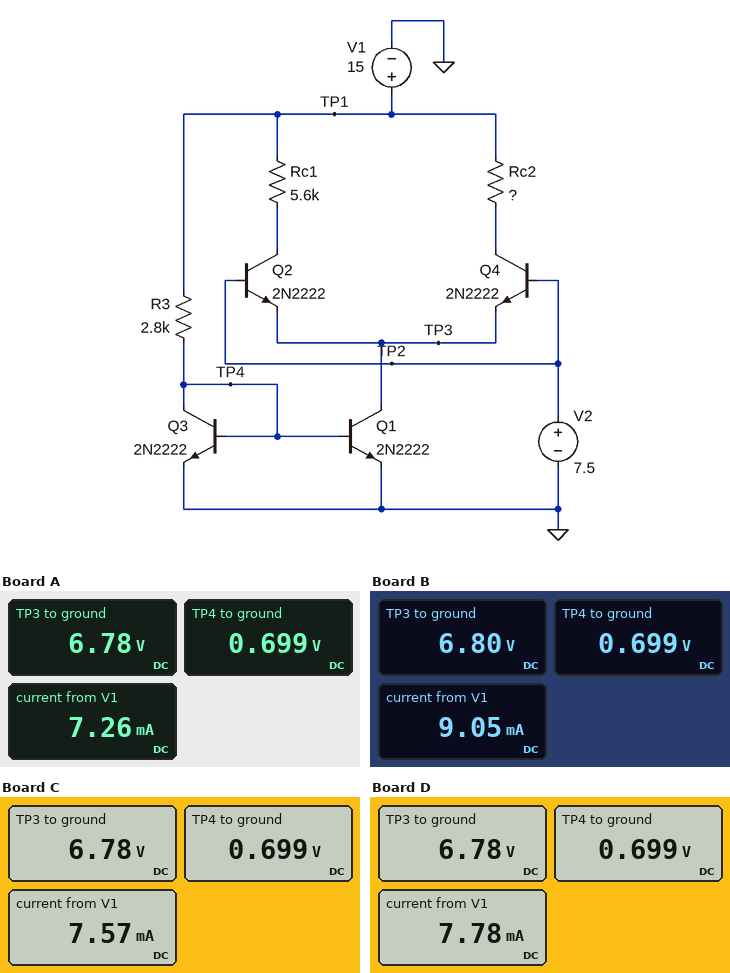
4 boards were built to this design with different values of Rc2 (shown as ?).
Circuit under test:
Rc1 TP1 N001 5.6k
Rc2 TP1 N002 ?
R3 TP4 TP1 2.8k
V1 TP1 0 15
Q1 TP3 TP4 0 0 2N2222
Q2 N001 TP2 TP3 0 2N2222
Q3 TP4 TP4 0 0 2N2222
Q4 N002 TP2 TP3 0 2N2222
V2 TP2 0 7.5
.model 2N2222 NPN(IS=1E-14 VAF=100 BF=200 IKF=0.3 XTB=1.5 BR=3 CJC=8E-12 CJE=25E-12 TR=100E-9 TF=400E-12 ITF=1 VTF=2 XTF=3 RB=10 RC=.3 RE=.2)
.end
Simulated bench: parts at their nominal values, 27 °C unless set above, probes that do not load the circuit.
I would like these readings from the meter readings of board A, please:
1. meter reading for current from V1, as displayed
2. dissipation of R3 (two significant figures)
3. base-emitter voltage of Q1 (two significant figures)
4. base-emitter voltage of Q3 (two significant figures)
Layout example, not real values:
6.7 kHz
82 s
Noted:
7.26 mA
73 mW
700 mV
700 mV
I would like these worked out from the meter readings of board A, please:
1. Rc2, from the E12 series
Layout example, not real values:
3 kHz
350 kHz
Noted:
12 kΩ
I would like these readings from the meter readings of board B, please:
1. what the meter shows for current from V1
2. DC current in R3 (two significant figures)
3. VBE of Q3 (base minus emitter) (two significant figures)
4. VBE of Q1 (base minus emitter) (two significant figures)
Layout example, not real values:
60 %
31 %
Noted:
9.05 mA
5.1 mA
700 mV
700 mV
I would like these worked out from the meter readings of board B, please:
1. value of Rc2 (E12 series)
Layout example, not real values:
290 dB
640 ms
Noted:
3.3 kΩ
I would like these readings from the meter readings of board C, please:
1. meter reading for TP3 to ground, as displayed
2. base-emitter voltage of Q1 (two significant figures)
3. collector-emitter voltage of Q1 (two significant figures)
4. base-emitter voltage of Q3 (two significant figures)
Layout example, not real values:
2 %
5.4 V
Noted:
6.78 V
700 mV
6.8 V
700 mV
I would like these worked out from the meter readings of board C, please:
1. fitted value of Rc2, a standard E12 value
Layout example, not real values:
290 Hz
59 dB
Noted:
8.2 kΩ
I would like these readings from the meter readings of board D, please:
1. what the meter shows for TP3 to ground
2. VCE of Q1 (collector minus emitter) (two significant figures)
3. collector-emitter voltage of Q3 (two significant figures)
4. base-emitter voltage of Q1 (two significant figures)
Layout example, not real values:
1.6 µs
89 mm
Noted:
6.78 V
6.8 V
700 mV
700 mV
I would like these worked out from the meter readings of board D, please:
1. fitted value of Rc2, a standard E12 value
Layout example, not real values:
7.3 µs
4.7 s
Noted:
6.8 kΩ
